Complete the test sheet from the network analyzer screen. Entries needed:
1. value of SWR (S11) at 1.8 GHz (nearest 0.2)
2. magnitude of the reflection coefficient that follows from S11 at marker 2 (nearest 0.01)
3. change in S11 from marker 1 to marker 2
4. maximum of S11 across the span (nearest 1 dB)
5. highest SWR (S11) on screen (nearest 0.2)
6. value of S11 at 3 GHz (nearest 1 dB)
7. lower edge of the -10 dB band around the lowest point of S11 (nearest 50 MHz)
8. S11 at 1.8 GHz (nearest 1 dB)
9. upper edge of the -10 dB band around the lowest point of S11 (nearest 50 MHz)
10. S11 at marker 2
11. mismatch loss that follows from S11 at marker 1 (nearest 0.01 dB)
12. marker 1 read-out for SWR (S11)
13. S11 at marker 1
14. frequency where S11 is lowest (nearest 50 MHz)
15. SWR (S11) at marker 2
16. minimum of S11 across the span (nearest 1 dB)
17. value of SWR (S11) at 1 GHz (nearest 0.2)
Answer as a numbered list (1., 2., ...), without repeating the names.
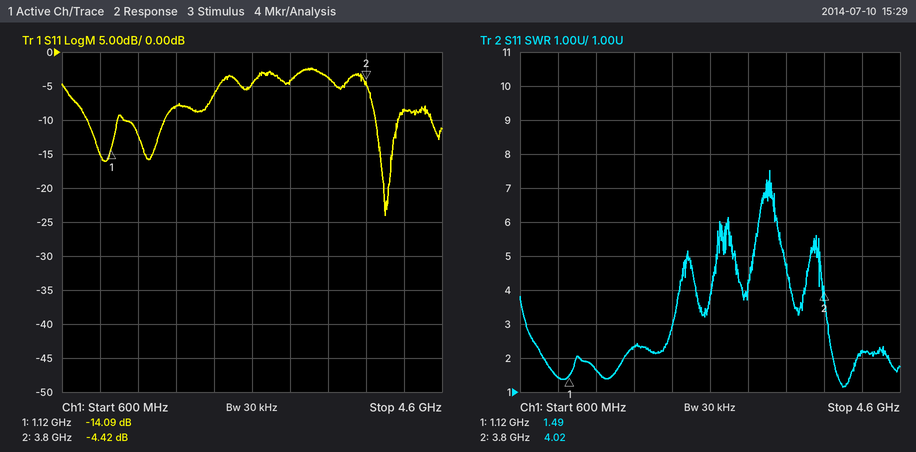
1. 2.4
2. 0.60
3. 9.67 dB
4. -2 dB
5. 7.6
6. -4 dB
7. 3.90 GHz
8. -8 dB
9. 4.15 GHz
10. -4.42 dB
11. 0.17 dB
12. 1.49
13. -14.09 dB
14. 4.00 GHz
15. 4.02
16. -24 dB
17. 1.4
